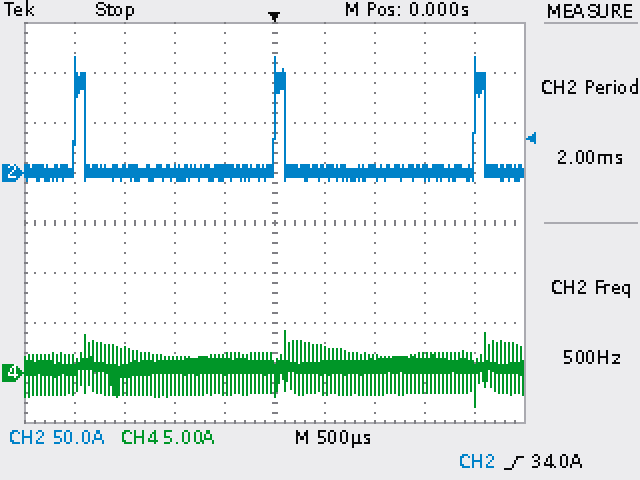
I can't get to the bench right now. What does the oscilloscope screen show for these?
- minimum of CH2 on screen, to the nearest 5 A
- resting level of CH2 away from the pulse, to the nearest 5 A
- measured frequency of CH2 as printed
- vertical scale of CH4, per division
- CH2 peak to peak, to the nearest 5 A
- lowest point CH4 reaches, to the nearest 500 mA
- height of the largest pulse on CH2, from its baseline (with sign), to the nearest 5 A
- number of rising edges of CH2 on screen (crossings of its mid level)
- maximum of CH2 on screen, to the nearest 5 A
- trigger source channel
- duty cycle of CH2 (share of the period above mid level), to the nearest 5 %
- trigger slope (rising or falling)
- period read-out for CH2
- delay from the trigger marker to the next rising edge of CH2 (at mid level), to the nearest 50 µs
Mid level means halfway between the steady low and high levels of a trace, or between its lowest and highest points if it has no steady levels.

-10 A
0 A
500 Hz
5 A
125 A
-3.5 A
+115 A
3
115 A
CH2
5 %
rising
2.00 ms
2.00 ms
